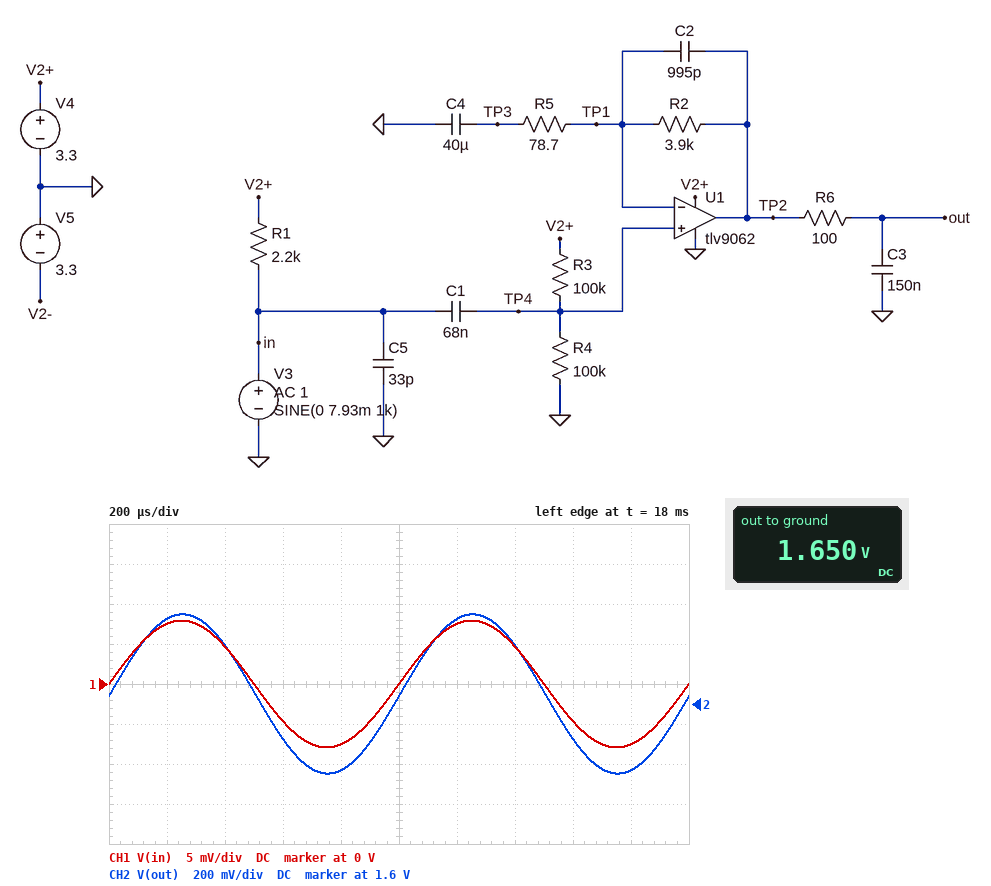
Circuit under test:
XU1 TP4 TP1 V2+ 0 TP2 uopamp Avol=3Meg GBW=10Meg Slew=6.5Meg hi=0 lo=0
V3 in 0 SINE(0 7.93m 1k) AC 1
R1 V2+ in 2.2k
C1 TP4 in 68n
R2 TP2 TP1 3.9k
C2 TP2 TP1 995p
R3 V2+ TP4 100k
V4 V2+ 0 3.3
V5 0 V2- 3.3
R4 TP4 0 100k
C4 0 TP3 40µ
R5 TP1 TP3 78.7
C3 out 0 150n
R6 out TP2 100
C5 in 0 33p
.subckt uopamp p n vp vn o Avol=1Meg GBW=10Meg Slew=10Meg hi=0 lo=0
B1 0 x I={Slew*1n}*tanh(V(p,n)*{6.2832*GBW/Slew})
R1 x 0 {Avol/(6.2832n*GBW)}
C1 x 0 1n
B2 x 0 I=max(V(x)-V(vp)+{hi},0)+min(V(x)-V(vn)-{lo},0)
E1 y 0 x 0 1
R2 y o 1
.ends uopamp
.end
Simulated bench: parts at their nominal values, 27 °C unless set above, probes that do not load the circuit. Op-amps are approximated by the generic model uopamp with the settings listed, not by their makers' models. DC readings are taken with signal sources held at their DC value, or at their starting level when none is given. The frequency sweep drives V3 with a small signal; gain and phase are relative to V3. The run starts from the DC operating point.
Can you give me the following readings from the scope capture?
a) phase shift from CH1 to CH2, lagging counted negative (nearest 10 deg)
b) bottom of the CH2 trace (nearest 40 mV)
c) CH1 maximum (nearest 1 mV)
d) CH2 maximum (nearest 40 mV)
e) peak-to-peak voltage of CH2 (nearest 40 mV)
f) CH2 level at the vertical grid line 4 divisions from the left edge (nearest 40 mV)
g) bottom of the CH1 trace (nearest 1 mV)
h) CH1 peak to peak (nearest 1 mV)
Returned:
0 deg
1.24 V
8 mV
2.04 V
800 mV
1.28 V
-8 mV
16 mV
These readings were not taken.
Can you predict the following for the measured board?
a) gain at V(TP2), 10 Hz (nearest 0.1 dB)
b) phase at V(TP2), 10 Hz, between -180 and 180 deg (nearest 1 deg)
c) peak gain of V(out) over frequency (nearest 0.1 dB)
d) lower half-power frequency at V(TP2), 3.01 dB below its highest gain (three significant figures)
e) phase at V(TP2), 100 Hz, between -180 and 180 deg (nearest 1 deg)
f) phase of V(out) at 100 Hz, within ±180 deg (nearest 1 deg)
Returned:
6.3 dB
151 deg
34.0 dB
75.4 Hz
51 deg
51 deg
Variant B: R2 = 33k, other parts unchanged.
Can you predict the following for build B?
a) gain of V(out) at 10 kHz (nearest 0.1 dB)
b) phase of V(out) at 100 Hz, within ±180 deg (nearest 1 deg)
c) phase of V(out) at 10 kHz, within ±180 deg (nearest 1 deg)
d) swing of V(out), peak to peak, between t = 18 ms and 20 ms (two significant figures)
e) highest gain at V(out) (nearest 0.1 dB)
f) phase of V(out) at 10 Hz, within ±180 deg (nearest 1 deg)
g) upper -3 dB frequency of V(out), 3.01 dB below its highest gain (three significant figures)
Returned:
41.2 dB
50 deg
-111 deg
3.3 V
52.3 dB
156 deg
3.70 kHz
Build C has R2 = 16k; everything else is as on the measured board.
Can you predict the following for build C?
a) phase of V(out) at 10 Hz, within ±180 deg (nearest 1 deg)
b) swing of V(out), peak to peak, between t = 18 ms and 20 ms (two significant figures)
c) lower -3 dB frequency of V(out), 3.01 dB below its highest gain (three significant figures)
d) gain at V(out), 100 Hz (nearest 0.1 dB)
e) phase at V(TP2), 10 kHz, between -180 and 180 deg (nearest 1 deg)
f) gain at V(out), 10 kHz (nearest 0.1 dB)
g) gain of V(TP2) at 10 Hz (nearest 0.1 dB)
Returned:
155 deg
3.2 V
74.4 Hz
44.4 dB
-50 deg
39.6 dB
18.4 dB
